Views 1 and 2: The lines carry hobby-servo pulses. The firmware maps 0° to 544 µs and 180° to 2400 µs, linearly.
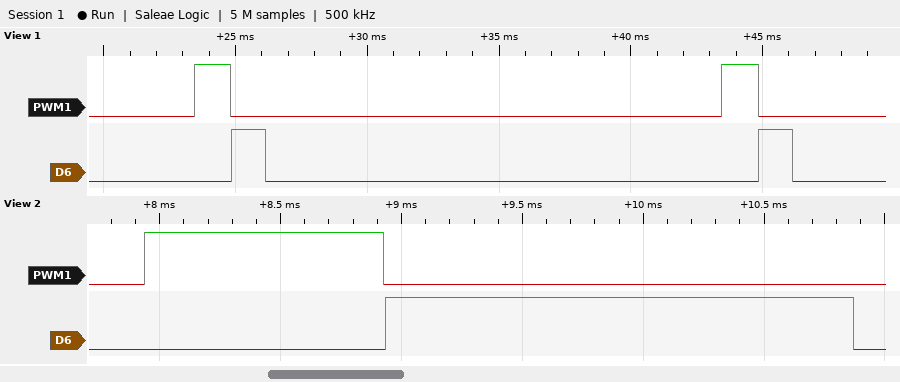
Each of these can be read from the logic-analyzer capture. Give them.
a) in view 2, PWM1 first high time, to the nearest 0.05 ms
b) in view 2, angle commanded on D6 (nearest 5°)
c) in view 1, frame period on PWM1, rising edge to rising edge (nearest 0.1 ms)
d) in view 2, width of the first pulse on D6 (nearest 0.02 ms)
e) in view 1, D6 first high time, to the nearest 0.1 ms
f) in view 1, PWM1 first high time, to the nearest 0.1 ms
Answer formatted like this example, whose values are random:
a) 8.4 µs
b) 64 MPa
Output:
a) 1.00 ms
b) 135°
c) 20.0 ms
d) 1.94 ms
e) 1.3 ms
f) 1.4 ms
